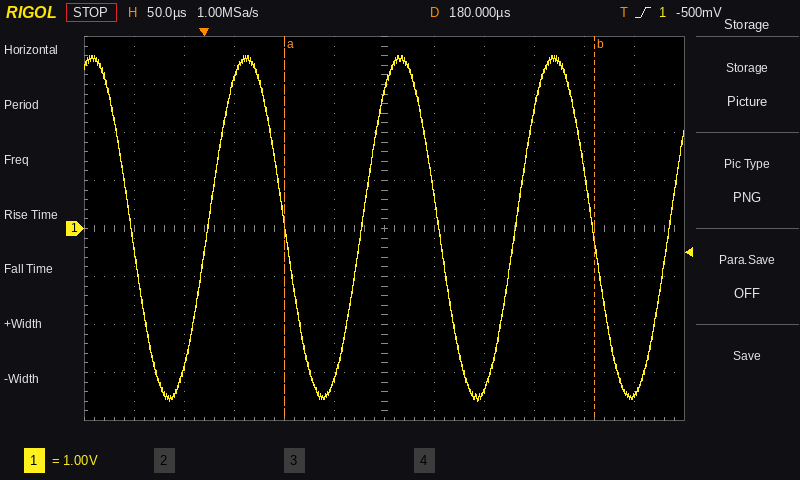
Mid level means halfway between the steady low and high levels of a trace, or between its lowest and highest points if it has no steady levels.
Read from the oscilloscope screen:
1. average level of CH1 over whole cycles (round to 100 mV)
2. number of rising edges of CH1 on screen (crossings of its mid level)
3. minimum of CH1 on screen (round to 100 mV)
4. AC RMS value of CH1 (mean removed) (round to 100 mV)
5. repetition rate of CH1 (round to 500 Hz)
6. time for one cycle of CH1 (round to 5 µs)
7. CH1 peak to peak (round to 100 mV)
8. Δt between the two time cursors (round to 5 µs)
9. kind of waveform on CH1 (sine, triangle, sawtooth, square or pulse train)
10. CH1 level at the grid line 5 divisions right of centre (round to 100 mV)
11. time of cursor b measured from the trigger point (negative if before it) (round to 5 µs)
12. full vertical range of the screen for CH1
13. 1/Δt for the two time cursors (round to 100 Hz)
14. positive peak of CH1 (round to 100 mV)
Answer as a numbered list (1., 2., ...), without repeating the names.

1. 0.0 V
2. 4
3. -3.6 V
4. 2.5 V
5. 6.5 kHz
6. 155 µs
7. 7.2 V
8. 310 µs
9. sine
10. -3.5 V
11. +390 µs
12. 8 V
13. 3.2 kHz
14. 3.6 V
